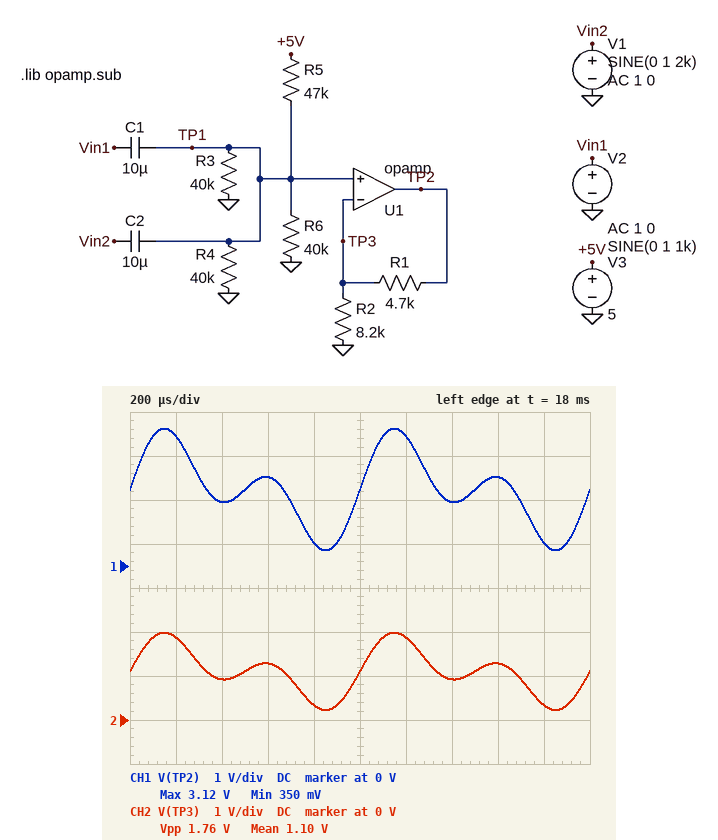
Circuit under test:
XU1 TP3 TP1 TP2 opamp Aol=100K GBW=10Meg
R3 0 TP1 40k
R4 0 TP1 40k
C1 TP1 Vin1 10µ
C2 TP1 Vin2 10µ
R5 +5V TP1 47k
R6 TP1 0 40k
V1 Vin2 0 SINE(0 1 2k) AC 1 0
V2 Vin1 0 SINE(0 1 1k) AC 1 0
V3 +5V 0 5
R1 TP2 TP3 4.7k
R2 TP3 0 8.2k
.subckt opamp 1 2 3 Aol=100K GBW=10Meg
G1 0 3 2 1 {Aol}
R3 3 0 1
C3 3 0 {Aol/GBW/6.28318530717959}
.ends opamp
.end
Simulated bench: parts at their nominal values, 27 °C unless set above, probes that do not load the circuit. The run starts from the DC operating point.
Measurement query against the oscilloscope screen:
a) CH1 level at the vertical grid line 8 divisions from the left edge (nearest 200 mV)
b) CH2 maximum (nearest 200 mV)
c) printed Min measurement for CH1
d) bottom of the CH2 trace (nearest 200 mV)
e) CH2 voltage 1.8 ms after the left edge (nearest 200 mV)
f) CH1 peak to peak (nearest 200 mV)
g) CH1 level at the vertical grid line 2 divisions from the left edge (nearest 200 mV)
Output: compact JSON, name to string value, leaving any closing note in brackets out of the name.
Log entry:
{"CH1 level at the vertical grid line 8 divisions from the left edge": "2.0 V", "CH2 maximum": "2.0 V", "printed Min measurement for CH1": "350 mV", "bottom of the CH2 trace": "200 mV", "CH2 voltage 1.8 ms after the left edge": "400 mV", "CH1 peak to peak": "2.8 V", "CH1 level at the vertical grid line 2 divisions from the left edge": "1.4 V"}
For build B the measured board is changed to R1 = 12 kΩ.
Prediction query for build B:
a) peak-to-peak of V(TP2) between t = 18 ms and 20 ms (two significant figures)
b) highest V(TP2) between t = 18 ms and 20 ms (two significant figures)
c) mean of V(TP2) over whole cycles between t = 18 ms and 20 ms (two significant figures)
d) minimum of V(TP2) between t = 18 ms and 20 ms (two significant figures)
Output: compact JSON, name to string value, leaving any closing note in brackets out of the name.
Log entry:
{"peak-to-peak of V(TP2) between t = 18 ms and 20 ms": "4.3 V", "highest V(TP2) between t = 18 ms and 20 ms": "4.9 V", "mean of V(TP2) over whole cycles between t = 18 ms and 20 ms": "2.7 V", "minimum of V(TP2) between t = 18 ms and 20 ms": "550 mV"}
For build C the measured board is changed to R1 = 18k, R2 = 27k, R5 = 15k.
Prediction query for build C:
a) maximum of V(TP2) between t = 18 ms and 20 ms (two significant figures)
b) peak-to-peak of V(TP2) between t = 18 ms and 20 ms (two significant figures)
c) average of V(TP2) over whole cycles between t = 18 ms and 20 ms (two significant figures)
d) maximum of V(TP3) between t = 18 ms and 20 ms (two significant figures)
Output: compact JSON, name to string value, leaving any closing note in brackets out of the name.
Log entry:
{"maximum of V(TP2) between t = 18 ms and 20 ms": "5.4 V", "peak-to-peak of V(TP2) between t = 18 ms and 20 ms": "2.9 V", "average of V(TP2) over whole cycles between t = 18 ms and 20 ms": "3.9 V", "maximum of V(TP3) between t = 18 ms and 20 ms": "3.2 V"}
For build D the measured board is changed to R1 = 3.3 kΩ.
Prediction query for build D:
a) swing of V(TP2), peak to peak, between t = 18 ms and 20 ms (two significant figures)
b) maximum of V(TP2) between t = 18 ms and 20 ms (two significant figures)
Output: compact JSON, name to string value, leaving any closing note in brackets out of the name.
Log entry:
{"swing of V(TP2), peak to peak, between t = 18 ms and 20 ms": "2.5 V", "maximum of V(TP2) between t = 18 ms and 20 ms": "2.8 V"}
